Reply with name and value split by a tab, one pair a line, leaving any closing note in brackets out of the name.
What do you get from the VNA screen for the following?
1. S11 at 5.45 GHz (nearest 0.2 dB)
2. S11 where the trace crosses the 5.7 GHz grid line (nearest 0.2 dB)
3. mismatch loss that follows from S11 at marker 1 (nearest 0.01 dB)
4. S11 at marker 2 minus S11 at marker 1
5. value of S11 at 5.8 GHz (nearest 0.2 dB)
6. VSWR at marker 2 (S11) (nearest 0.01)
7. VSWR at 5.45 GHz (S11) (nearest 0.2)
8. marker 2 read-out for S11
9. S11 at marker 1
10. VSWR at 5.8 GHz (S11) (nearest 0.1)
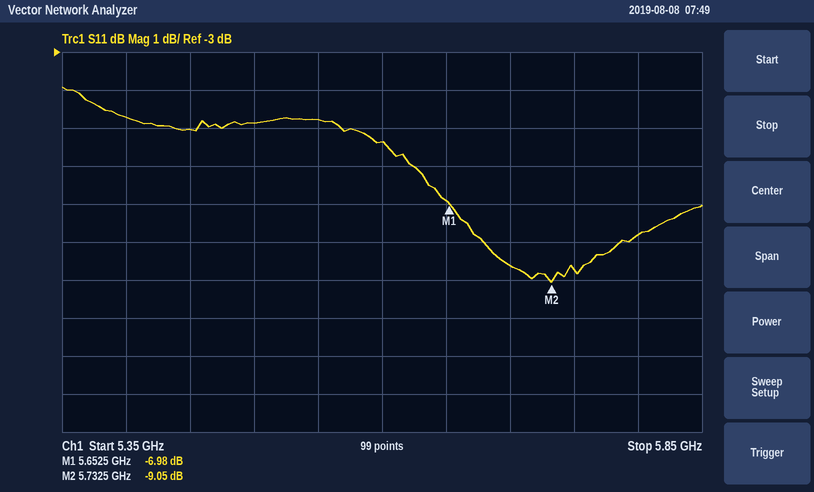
S11 at 5.45 GHz	-5.0 dB
S11 where the trace crosses the 5.7 GHz grid line	-8.6 dB
mismatch loss that follows from S11 at marker 1	0.97 dB
S11 at marker 2 minus S11 at marker 1	-2.07 dB
value of S11 at 5.8 GHz	-7.8 dB
VSWR at marker 2 (S11)	2.09
VSWR at 5.45 GHz (S11)	3.6
marker 2 read-out for S11	-9.05 dB
S11 at marker 1	-6.98 dB
VSWR at 5.8 GHz (S11)	2.4
